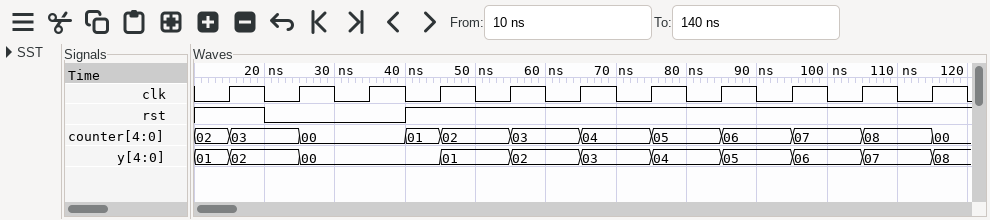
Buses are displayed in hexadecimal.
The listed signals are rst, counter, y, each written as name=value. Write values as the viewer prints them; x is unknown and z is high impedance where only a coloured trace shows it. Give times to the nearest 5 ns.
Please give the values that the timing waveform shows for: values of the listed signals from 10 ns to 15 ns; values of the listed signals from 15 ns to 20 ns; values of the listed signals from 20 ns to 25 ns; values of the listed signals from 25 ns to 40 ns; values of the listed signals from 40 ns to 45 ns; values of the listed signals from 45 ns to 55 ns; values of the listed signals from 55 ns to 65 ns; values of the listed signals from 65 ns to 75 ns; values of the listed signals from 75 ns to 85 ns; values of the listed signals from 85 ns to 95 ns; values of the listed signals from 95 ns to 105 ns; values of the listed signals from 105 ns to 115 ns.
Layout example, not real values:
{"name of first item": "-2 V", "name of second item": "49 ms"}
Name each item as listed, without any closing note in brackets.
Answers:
{"values of the listed signals from 10 ns to 15 ns": "rst=1, counter=02, y=01", "values of the listed signals from 15 ns to 20 ns": "rst=1, counter=03, y=02", "values of the listed signals from 20 ns to 25 ns": "rst=0, counter=03, y=02", "values of the listed signals from 25 ns to 40 ns": "rst=0, counter=00, y=00", "values of the listed signals from 40 ns to 45 ns": "rst=1, counter=01, y=00", "values of the listed signals from 45 ns to 55 ns": "rst=1, counter=02, y=01", "values of the listed signals from 55 ns to 65 ns": "rst=1, counter=03, y=02", "values of the listed signals from 65 ns to 75 ns": "rst=1, counter=04, y=03", "values of the listed signals from 75 ns to 85 ns": "rst=1, counter=05, y=04", "values of the listed signals from 85 ns to 95 ns": "rst=1, counter=06, y=05", "values of the listed signals from 95 ns to 105 ns": "rst=1, counter=07, y=06", "values of the listed signals from 105 ns to 115 ns": "rst=1, counter=08, y=07"}
